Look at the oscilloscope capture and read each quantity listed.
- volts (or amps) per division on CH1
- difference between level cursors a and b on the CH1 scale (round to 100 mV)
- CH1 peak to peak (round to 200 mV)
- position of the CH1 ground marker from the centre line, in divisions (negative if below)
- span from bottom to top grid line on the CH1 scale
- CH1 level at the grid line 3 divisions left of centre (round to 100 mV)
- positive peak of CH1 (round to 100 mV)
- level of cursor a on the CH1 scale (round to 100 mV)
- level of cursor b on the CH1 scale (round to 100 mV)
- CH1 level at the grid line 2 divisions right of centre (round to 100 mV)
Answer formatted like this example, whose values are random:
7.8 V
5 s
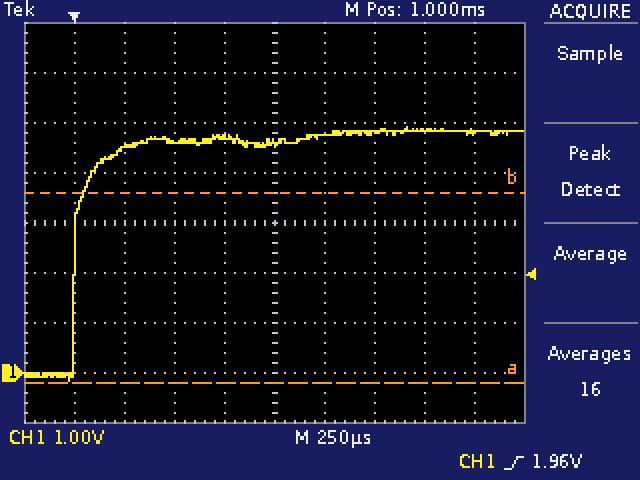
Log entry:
1 V
3.8 V
5.0 V
-3.0 div
8 V
4.5 V
4.9 V
-200 mV
3.6 V
4.8 V
